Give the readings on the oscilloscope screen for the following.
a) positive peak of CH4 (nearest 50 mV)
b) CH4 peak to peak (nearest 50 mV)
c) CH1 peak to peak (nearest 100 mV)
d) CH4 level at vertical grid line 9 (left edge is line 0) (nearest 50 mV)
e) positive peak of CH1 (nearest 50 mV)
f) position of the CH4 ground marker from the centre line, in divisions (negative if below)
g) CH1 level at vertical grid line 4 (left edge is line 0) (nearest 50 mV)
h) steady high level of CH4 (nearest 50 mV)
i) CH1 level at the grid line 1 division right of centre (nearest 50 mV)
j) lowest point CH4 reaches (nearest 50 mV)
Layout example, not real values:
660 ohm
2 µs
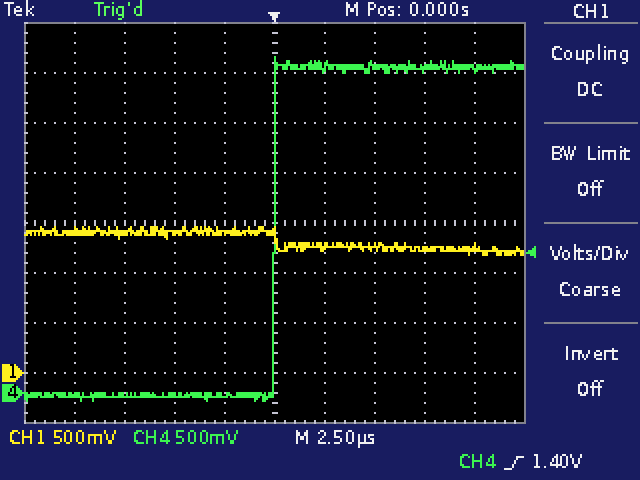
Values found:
3.35 V
3.45 V
300 mV
3.25 V
1.45 V
-3.4 div
1.40 V
3.25 V
1.25 V
-100 mV
